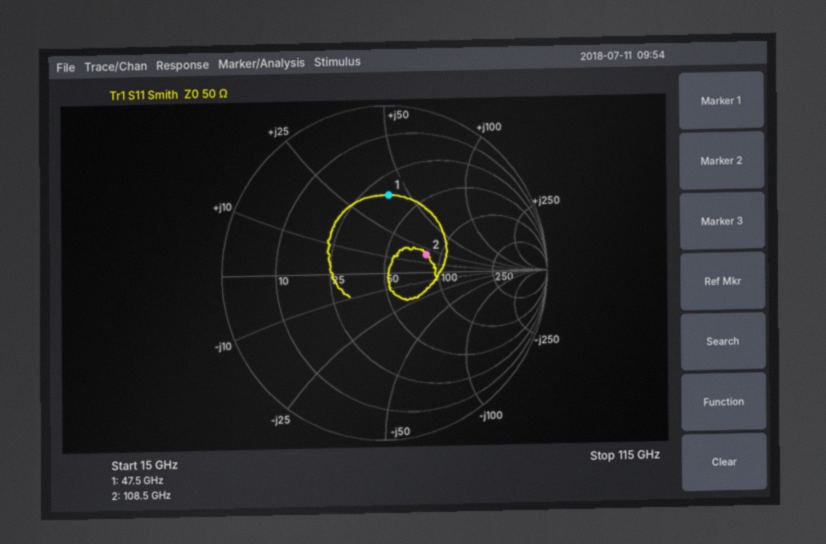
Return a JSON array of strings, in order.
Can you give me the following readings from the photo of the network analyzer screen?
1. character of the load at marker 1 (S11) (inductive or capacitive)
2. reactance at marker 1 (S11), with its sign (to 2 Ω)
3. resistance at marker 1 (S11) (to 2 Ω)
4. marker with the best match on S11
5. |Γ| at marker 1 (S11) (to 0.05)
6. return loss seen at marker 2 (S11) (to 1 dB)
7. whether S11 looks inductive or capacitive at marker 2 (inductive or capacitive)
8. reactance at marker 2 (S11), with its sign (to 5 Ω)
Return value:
["inductive", "+40 Ω", "34 Ω", "marker 2", "0.45", "11 dB", "inductive", "+20 Ω"]
